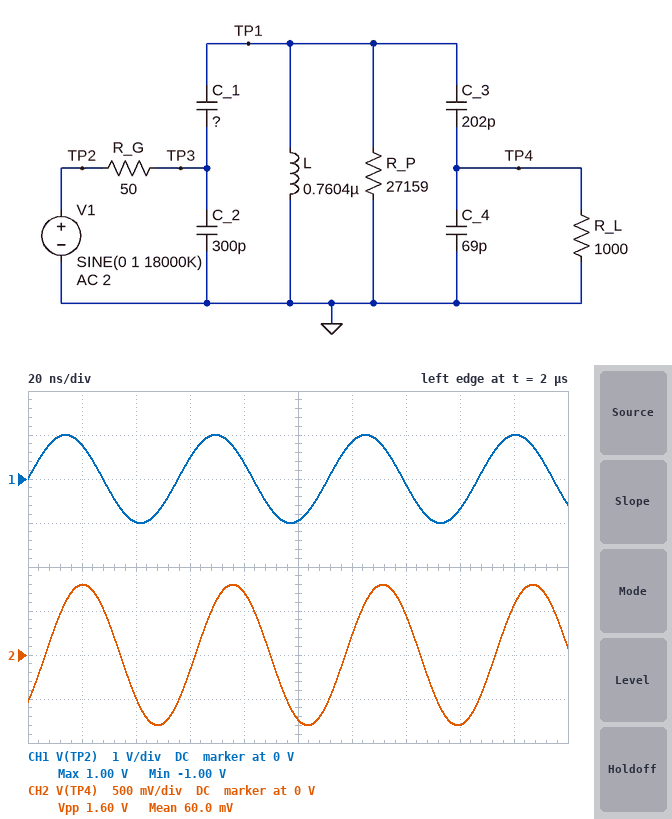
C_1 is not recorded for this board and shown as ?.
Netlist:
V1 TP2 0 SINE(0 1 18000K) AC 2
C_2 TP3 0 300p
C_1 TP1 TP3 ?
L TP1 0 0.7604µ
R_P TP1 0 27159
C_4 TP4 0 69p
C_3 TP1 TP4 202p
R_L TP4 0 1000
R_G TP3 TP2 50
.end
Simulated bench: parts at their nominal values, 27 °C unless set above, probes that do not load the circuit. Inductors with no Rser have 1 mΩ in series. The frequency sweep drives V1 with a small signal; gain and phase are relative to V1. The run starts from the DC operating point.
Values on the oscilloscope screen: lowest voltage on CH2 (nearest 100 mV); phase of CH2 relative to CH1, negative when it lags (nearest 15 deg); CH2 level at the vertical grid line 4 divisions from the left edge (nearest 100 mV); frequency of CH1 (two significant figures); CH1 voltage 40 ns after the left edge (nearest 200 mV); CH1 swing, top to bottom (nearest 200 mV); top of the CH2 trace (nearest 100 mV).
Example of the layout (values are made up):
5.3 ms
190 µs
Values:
-800 mV
-45 deg
700 mV
18 MHz
-1.0 V
2.0 V
800 mV
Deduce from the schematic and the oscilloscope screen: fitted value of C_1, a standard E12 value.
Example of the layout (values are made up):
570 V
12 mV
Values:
120 pF
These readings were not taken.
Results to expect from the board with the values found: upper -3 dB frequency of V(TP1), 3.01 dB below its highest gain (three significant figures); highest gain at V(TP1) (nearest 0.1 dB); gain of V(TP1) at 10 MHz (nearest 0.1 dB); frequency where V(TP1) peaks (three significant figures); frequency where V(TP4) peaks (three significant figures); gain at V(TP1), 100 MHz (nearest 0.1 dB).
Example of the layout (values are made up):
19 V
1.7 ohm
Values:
16.3 MHz
8.6 dB
-8.1 dB
15.2 MHz
15.2 MHz
-23.4 dB
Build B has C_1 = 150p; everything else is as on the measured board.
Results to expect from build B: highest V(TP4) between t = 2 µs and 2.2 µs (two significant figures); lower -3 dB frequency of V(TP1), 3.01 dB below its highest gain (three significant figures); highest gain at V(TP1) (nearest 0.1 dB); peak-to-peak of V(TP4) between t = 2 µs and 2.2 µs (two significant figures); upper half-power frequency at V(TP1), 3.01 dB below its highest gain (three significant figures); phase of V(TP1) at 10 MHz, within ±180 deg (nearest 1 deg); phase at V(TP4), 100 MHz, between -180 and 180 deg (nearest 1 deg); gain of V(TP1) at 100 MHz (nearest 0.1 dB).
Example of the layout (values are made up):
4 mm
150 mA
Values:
680 mV
13.2 MHz
8.0 dB
1.4 V
15.7 MHz
114 deg
-84 deg
-22.9 dB
